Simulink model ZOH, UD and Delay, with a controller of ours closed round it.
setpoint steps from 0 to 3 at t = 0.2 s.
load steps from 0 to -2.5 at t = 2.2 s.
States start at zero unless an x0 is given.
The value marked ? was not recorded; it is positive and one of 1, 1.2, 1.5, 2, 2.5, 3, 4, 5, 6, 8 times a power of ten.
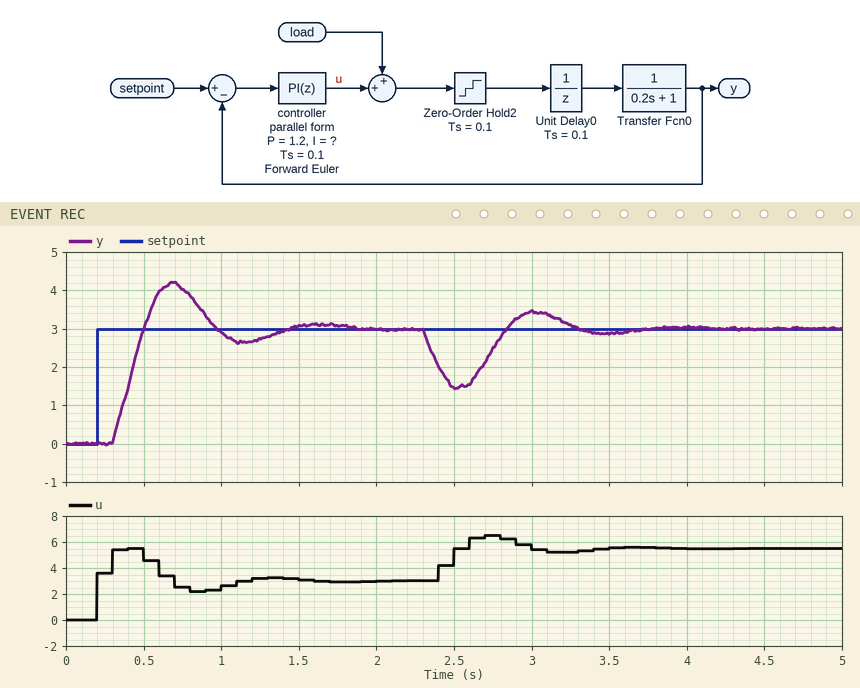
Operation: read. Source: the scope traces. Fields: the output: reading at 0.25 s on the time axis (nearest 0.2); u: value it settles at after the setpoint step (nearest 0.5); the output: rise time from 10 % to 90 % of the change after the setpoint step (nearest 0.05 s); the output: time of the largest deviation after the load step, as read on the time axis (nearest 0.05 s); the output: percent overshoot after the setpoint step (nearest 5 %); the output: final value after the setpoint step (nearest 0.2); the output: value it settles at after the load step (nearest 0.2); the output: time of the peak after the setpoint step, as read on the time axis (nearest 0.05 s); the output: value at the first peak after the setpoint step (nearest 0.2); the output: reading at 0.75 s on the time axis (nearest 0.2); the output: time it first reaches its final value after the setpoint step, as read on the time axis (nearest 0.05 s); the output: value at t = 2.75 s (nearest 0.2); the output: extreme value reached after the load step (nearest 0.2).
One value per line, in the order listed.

0.0
3.0
0.15 s
2.50 s
40 %
3.0
3.0
0.70 s
4.2
4.0
0.50 s
2.4
1.4
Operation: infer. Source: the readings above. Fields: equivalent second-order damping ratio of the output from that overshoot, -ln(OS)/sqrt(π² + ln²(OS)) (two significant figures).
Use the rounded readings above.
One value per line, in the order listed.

0.28
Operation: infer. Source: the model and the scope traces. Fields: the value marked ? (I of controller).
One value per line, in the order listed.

6
